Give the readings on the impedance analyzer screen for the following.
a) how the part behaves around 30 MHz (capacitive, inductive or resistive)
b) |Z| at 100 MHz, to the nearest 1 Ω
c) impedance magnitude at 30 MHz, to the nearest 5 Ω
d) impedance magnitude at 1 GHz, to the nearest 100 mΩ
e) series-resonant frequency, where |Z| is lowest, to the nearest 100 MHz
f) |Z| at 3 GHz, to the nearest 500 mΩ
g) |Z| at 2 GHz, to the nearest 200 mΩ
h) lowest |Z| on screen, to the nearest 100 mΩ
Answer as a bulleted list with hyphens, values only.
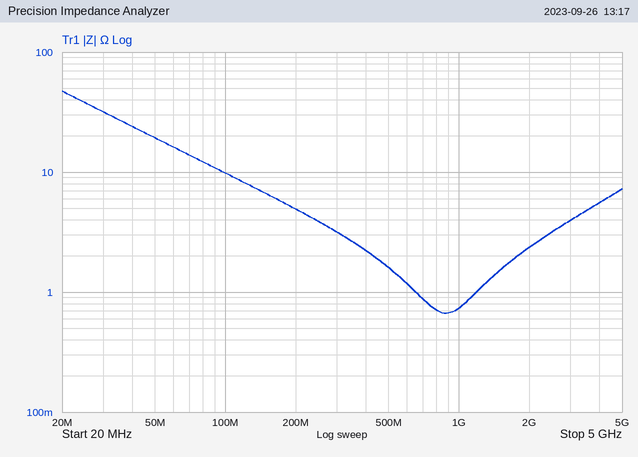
- capacitive
- 10 Ω
- 30 Ω
- 700 mΩ
- 900 MHz
- 4.0 Ω
- 2.4 Ω
- 700 mΩ
